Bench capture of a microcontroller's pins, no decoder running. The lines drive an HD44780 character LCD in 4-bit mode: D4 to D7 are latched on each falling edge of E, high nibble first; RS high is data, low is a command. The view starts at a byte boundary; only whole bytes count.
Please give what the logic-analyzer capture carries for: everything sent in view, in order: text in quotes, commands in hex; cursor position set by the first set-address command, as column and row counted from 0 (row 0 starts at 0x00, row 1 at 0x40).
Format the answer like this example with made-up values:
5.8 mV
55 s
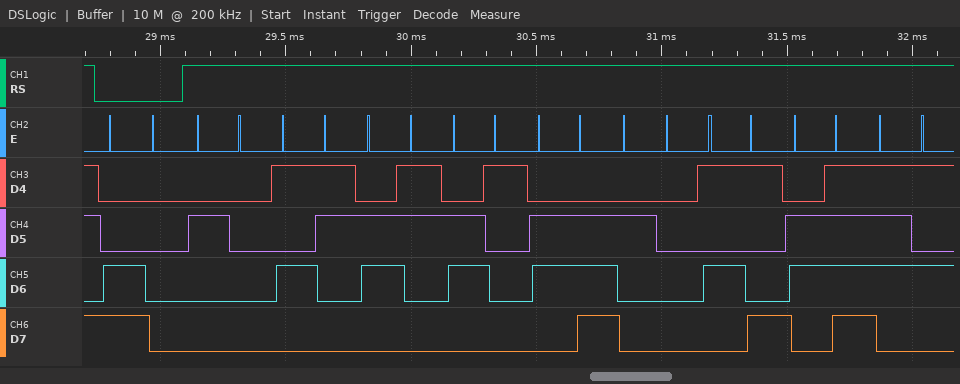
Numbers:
0xC0 " Scan You"
column 0, row 1
